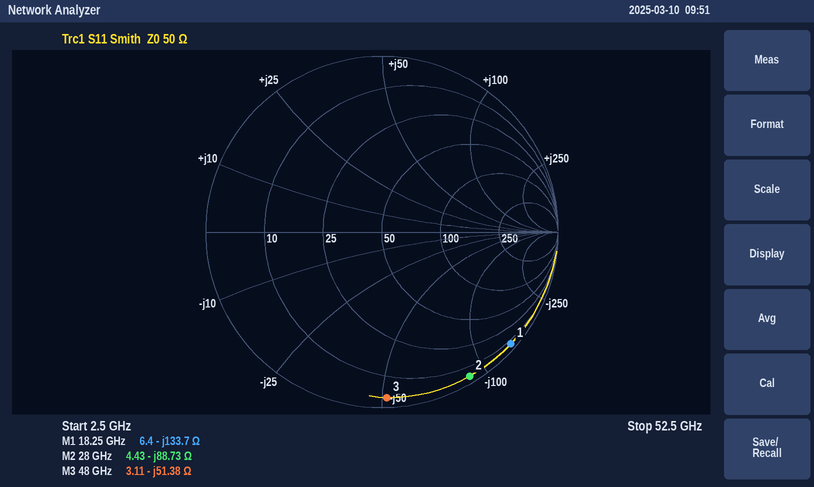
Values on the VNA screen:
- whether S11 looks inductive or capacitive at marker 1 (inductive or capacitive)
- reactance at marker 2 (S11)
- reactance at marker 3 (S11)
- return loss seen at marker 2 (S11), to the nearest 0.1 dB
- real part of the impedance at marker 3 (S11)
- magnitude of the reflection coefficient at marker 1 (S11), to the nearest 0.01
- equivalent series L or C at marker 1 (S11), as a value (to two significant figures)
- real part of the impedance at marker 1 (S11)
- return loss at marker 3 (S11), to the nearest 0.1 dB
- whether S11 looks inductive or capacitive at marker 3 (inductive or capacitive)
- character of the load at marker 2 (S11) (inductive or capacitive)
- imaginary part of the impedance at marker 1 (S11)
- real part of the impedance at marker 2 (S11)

capacitive
-88.73 Ω
-51.38 Ω
0.4 dB
3.11 Ω
0.97
65 fF
6.4 Ω
0.5 dB
capacitive
capacitive
-133.7 Ω
4.43 Ω
